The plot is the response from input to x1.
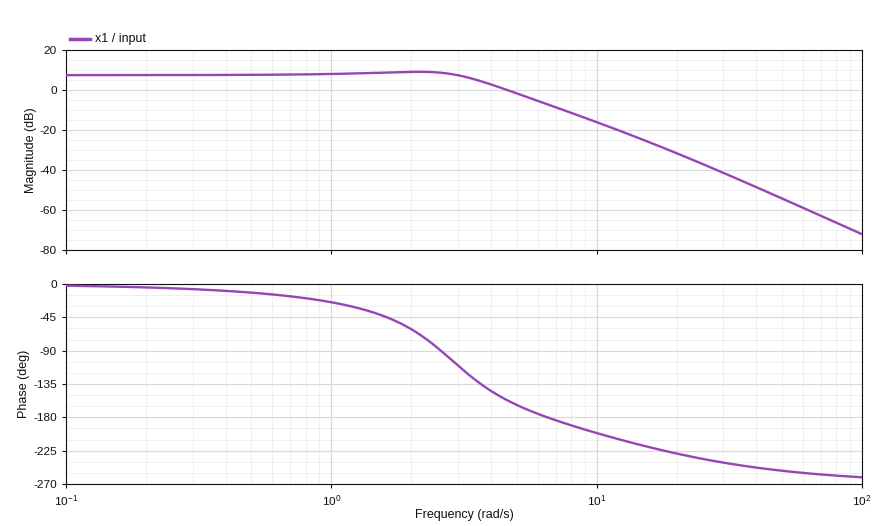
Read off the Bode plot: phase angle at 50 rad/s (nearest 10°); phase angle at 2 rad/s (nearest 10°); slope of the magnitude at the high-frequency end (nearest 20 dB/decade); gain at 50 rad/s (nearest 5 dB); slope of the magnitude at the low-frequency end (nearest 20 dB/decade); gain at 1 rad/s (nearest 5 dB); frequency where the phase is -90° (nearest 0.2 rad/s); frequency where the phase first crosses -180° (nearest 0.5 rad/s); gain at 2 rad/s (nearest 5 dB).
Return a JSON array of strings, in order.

["-250°", "-60°", "-60 dB/decade", "-55 dB", "0 dB/decade", "10 dB", "2.6 rad/s", "6.5 rad/s", "10 dB"]
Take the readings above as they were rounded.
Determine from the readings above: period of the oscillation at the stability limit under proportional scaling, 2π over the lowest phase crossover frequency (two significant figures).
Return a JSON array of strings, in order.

["0.97 s"]
